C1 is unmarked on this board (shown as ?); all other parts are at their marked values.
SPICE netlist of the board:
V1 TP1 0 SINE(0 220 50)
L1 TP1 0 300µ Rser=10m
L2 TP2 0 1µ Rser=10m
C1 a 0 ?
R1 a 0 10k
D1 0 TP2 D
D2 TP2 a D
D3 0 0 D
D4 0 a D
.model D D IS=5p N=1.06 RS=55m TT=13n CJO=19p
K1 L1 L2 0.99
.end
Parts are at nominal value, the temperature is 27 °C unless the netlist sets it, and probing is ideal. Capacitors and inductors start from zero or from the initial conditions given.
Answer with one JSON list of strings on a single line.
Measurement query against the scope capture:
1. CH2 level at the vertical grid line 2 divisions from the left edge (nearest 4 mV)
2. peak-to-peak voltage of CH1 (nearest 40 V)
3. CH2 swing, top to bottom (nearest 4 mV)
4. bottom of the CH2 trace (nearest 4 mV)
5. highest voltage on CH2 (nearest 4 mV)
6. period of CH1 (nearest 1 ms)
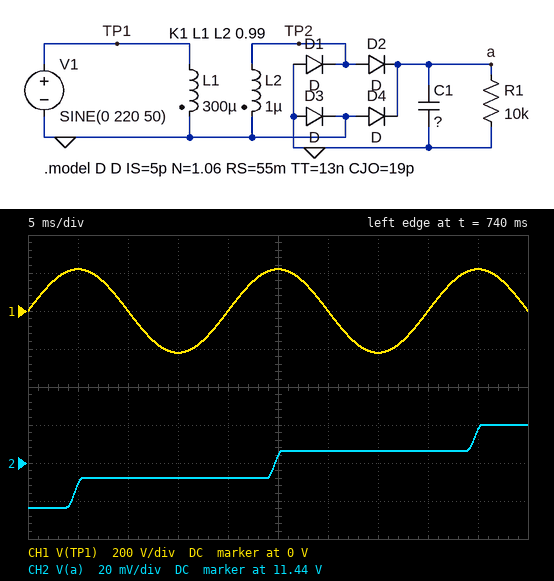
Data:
["11.432 V", "440 V", "44 mV", "11.416 V", "11.460 V", "20 ms"]
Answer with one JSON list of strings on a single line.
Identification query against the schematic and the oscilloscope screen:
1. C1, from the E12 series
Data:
["330 mF"]
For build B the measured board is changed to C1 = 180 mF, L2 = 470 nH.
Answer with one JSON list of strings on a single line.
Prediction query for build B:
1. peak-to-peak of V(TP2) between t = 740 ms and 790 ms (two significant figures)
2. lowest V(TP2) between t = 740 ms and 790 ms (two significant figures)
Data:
["16 V", "-7.4 V"]
